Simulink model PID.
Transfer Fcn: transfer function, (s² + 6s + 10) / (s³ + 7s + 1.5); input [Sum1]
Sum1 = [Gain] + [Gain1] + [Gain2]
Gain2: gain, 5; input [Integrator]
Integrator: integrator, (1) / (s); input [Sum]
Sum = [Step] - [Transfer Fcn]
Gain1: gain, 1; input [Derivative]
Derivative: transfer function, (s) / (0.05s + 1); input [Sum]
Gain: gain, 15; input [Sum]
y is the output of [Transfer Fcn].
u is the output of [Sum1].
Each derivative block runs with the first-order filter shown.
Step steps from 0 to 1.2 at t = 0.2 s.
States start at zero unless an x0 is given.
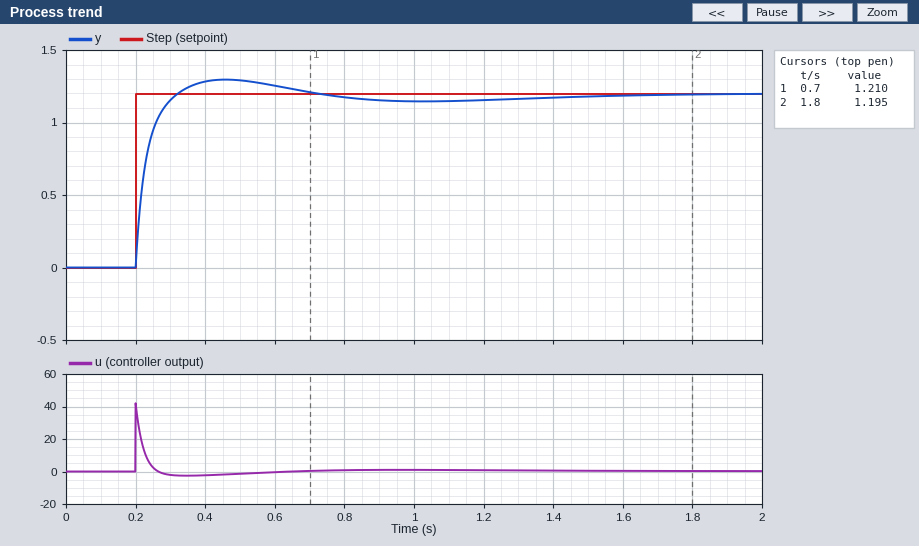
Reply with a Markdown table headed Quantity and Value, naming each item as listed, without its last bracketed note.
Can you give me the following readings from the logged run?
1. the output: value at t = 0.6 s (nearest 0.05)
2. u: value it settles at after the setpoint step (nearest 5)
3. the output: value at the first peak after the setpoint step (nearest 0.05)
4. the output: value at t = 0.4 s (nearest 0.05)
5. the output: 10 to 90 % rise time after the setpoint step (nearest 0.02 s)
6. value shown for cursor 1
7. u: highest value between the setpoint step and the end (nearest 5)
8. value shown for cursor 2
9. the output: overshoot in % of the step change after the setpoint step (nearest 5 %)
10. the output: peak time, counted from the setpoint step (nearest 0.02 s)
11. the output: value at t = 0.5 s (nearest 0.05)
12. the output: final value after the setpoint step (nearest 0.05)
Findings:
| Quantity | Value |
|---|---|
| the output: value at t = 0.6 s | 1.25 |
| u: value it settles at after the setpoint step | 0 |
| the output: value at the first peak after the setpoint step | 1.30 |
| the output: value at t = 0.4 s | 1.30 |
| the output: 10 to 90 % rise time after the setpoint step | 0.08 s |
| value shown for cursor 1 | 1.210 |
| u: highest value between the setpoint step and the end | 40 |
| value shown for cursor 2 | 1.195 |
| the output: overshoot in % of the step change after the setpoint step | 10 % |
| the output: peak time, counted from the setpoint step | 0.26 s |
| the output: value at t = 0.5 s | 1.30 |
| the output: final value after the setpoint step | 1.20 |
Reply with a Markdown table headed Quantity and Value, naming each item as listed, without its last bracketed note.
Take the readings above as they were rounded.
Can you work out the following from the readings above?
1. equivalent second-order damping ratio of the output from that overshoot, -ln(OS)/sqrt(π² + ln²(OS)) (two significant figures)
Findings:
| Quantity | Value |
|---|---|
| equivalent second-order damping ratio of the output from that overshoot, -ln(OS)/sqrt(π² + ln²(OS)) | 0.59 |
